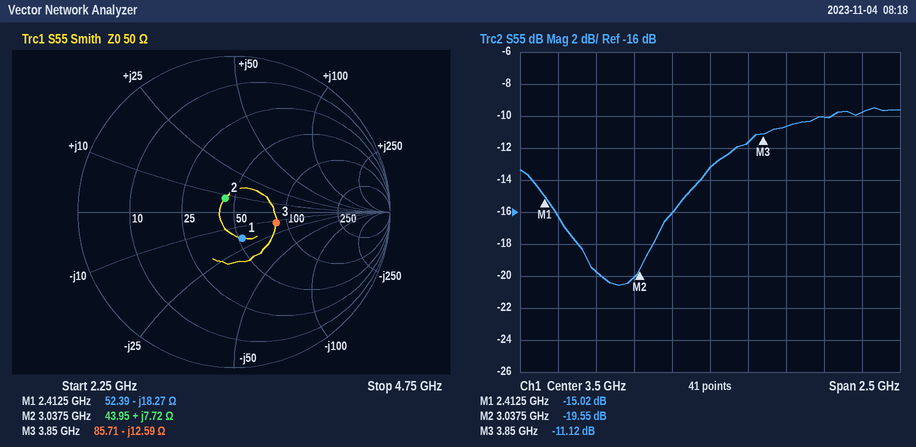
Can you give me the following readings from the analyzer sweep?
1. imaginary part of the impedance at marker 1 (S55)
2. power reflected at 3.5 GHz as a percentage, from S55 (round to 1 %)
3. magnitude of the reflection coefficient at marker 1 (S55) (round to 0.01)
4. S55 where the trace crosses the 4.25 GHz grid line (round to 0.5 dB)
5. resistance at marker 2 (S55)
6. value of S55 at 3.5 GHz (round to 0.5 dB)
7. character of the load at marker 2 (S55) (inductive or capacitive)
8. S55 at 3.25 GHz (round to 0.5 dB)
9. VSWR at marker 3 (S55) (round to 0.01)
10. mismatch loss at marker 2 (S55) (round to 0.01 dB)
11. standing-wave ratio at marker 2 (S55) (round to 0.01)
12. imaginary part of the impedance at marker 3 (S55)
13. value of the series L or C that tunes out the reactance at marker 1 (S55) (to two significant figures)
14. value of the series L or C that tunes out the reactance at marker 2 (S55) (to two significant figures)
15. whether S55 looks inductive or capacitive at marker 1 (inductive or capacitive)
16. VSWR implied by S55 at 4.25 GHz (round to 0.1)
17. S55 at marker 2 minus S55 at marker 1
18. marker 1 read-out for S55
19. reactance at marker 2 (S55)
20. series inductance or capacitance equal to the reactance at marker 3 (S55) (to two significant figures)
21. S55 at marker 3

-18.27 Ω
5 %
0.18
-10.0 dB
43.95 Ω
-13.0 dB
inductive
-16.0 dB
1.77
0.05 dB
1.23
-12.59 Ω
1.2 nH
6.8 pF
capacitive
1.9
-4.53 dB
-15.02 dB
+7.72 Ω
3.3 pF
-11.12 dB
